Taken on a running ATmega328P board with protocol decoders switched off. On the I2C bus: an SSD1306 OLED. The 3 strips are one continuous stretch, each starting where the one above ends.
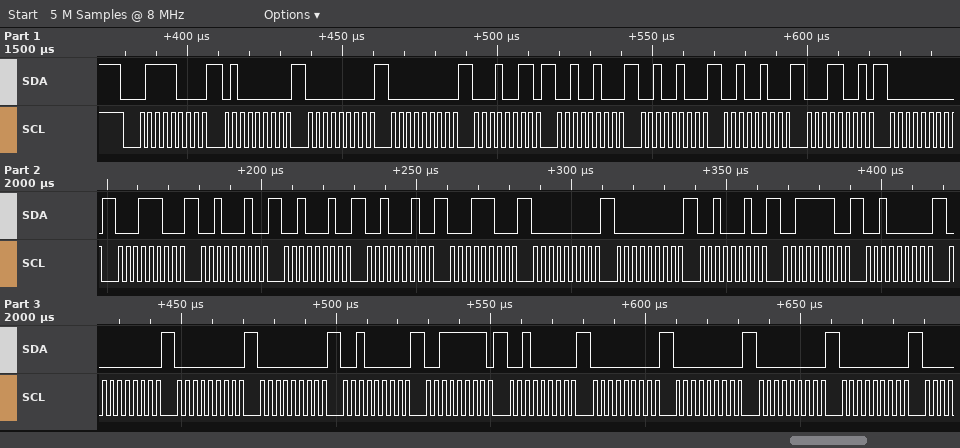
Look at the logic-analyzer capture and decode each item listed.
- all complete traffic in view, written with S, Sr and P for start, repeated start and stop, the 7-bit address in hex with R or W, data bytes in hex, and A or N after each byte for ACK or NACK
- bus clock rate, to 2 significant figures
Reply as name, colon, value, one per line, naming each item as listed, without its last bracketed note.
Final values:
all complete traffic in view, written with S, Sr and P for start, repeated start and stop, the 7-bit address in hex with R or W, data bytes in hex, and A or N after each byte for ACK or NACK: S 3CW A 40 A 00 A 00 A 13 A 24 A 24 A 24 A 19 A 00 A 1C A 22 A 22 A 22 A 1C A 00 A 00 A 22 A 3E A 20 A 00 A 00 A 00 A 20 A 3F A 20 A 00 A 00 A 00 A 00 A
bus clock rate, to 2 significant figures: 400 kHz
